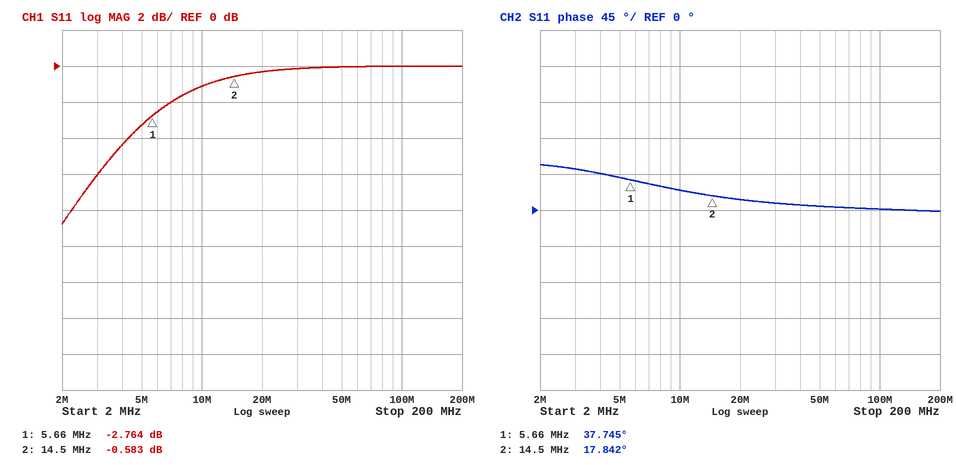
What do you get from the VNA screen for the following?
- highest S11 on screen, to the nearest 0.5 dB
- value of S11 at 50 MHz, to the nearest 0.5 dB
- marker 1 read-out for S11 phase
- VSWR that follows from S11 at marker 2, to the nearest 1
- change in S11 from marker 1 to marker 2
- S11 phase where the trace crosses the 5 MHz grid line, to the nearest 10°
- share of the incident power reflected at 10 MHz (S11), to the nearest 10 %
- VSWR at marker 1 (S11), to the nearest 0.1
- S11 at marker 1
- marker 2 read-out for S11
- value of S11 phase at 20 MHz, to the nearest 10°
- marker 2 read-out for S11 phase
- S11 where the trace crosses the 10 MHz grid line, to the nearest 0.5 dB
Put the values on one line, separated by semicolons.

0.0 dB; 0.0 dB; 37.745°; 30; 2.181 dB; 40°; 80 %; 6.3; -2.764 dB; -0.583 dB; 10°; 17.842°; -1.0 dB
